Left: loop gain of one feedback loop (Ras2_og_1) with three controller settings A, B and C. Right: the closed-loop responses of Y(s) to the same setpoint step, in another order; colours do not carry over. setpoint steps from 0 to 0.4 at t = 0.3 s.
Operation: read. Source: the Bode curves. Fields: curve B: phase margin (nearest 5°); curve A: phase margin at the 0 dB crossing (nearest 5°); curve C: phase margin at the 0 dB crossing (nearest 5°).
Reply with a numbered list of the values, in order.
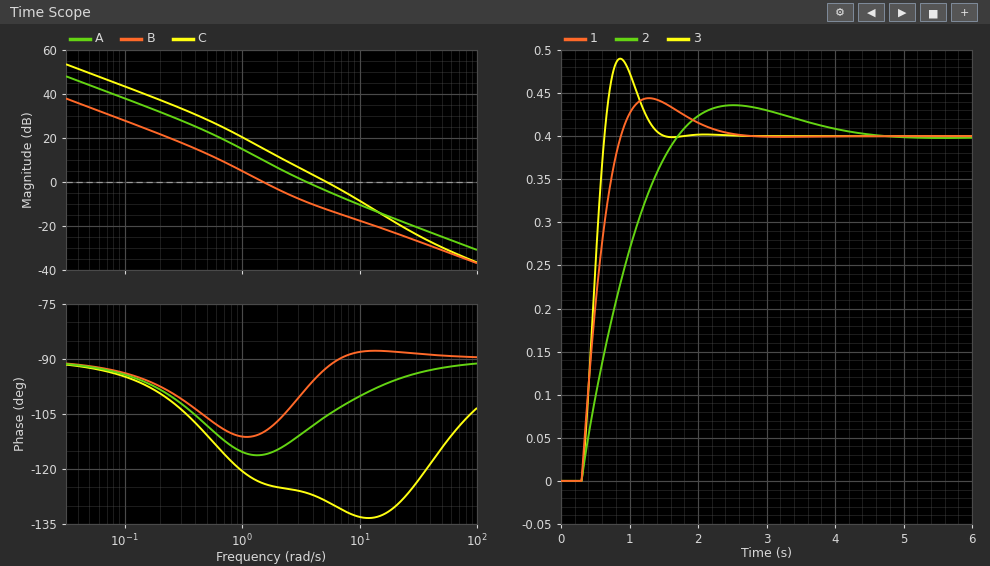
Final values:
1. 70°
2. 70°
3. 50°
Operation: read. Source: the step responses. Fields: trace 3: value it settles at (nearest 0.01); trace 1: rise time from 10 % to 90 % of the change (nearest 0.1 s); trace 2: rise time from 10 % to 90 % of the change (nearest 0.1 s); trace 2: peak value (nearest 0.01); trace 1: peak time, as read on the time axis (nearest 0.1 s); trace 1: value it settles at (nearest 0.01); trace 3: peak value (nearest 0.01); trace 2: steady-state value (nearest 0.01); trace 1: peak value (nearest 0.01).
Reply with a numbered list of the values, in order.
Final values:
1. 0.40
2. 0.4 s
3. 1.0 s
4. 0.44
5. 1.3 s
6. 0.40
7. 0.49
8. 0.40
9. 0.44
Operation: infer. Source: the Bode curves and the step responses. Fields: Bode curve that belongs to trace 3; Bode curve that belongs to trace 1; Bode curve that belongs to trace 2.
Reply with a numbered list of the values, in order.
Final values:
1. C
2. A
3. B
